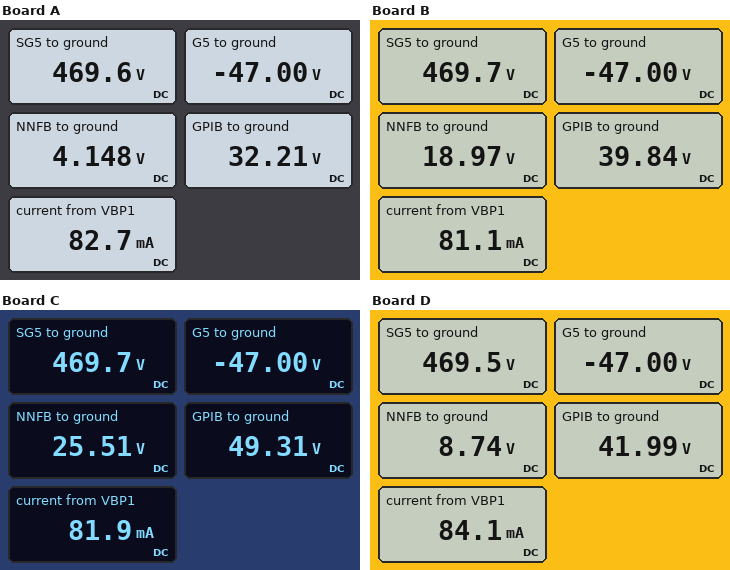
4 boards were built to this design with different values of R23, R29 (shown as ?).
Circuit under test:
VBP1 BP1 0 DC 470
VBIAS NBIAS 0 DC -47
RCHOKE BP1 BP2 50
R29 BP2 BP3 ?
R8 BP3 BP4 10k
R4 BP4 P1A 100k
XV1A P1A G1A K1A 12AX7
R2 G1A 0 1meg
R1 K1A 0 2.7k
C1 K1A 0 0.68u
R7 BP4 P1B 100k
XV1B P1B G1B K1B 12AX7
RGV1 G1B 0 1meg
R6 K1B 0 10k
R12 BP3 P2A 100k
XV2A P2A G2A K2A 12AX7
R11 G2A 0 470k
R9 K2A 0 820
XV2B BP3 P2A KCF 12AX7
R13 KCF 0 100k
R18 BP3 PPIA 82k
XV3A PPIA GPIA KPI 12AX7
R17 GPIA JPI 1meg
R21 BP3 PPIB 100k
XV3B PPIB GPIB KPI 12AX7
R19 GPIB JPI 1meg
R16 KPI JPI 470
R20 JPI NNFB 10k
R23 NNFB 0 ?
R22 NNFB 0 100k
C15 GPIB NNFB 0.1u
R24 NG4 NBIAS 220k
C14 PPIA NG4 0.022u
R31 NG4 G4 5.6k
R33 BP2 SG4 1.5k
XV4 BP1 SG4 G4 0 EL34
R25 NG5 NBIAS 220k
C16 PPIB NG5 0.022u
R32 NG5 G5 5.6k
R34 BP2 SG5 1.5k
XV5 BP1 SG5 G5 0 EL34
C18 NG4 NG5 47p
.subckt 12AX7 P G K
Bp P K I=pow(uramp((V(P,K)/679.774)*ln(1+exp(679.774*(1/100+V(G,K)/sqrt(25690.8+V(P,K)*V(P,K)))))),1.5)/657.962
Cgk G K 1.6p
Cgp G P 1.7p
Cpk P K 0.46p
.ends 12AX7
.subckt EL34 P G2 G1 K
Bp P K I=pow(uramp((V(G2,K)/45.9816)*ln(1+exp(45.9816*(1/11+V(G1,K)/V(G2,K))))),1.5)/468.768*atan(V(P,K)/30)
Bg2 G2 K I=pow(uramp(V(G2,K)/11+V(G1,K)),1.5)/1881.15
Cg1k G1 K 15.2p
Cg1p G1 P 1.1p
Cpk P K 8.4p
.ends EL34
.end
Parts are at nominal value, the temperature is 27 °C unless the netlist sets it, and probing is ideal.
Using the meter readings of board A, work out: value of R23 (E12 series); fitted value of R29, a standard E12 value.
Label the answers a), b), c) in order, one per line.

a) 1.5 kΩ
b) 15 kΩ
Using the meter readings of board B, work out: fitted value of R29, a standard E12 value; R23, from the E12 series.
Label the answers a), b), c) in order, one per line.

a) 33 kΩ
b) 10 kΩ
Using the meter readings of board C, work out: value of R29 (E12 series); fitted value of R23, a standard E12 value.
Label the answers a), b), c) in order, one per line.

a) 22 kΩ
b) 12 kΩ
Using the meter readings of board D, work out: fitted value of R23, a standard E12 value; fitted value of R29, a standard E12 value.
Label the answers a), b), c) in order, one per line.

a) 2.7 kΩ
b) 4.7 kΩ
